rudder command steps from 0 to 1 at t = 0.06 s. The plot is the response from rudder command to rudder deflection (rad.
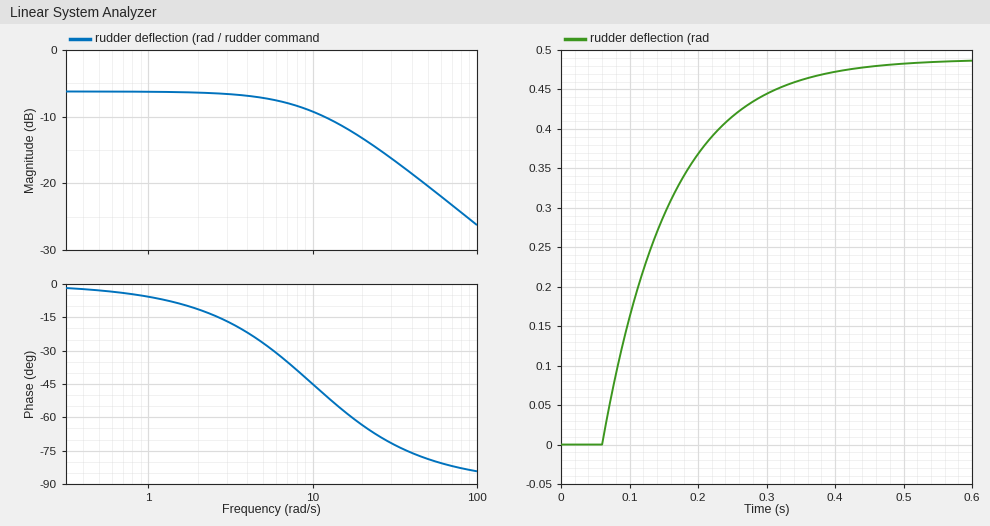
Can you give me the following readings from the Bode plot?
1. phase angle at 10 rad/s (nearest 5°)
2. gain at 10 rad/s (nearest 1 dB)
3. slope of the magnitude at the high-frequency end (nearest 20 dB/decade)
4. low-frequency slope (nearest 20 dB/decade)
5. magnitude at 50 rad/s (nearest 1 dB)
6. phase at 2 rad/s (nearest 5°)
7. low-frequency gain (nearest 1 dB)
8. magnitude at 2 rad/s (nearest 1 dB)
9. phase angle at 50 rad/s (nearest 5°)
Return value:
-45°
-9 dB
-20 dB/decade
0 dB/decade
-20 dB
-10°
-6 dB
-6 dB
-80°
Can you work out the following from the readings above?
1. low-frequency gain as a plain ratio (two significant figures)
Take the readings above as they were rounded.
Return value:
0.50
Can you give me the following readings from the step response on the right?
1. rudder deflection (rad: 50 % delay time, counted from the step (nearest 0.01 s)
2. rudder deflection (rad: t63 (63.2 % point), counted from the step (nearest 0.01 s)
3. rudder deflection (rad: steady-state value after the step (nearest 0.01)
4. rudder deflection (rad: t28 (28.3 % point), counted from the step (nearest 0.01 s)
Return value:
0.07 s
0.10 s
0.49
0.03 s
